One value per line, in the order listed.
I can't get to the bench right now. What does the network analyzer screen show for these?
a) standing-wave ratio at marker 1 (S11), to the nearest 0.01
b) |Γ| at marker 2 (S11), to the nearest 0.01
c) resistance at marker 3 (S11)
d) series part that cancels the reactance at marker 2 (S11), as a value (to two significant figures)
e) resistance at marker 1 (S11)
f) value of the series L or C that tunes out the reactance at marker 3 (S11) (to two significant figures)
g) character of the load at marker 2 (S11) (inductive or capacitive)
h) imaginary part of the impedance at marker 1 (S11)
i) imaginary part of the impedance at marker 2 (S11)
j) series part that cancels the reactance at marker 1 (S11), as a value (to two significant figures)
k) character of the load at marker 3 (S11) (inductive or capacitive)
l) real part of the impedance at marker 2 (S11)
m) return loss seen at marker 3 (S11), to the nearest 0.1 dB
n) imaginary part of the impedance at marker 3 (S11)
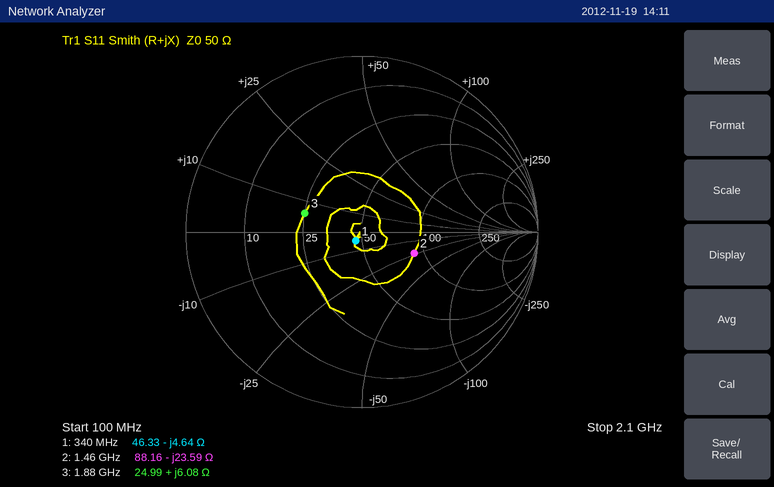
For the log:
1.13
0.32
24.99 Ω
2.6 nH
46.33 Ω
14 pF
capacitive
-4.64 Ω
-23.59 Ω
2.2 nH
inductive
88.16 Ω
9.3 dB
+6.08 Ω
